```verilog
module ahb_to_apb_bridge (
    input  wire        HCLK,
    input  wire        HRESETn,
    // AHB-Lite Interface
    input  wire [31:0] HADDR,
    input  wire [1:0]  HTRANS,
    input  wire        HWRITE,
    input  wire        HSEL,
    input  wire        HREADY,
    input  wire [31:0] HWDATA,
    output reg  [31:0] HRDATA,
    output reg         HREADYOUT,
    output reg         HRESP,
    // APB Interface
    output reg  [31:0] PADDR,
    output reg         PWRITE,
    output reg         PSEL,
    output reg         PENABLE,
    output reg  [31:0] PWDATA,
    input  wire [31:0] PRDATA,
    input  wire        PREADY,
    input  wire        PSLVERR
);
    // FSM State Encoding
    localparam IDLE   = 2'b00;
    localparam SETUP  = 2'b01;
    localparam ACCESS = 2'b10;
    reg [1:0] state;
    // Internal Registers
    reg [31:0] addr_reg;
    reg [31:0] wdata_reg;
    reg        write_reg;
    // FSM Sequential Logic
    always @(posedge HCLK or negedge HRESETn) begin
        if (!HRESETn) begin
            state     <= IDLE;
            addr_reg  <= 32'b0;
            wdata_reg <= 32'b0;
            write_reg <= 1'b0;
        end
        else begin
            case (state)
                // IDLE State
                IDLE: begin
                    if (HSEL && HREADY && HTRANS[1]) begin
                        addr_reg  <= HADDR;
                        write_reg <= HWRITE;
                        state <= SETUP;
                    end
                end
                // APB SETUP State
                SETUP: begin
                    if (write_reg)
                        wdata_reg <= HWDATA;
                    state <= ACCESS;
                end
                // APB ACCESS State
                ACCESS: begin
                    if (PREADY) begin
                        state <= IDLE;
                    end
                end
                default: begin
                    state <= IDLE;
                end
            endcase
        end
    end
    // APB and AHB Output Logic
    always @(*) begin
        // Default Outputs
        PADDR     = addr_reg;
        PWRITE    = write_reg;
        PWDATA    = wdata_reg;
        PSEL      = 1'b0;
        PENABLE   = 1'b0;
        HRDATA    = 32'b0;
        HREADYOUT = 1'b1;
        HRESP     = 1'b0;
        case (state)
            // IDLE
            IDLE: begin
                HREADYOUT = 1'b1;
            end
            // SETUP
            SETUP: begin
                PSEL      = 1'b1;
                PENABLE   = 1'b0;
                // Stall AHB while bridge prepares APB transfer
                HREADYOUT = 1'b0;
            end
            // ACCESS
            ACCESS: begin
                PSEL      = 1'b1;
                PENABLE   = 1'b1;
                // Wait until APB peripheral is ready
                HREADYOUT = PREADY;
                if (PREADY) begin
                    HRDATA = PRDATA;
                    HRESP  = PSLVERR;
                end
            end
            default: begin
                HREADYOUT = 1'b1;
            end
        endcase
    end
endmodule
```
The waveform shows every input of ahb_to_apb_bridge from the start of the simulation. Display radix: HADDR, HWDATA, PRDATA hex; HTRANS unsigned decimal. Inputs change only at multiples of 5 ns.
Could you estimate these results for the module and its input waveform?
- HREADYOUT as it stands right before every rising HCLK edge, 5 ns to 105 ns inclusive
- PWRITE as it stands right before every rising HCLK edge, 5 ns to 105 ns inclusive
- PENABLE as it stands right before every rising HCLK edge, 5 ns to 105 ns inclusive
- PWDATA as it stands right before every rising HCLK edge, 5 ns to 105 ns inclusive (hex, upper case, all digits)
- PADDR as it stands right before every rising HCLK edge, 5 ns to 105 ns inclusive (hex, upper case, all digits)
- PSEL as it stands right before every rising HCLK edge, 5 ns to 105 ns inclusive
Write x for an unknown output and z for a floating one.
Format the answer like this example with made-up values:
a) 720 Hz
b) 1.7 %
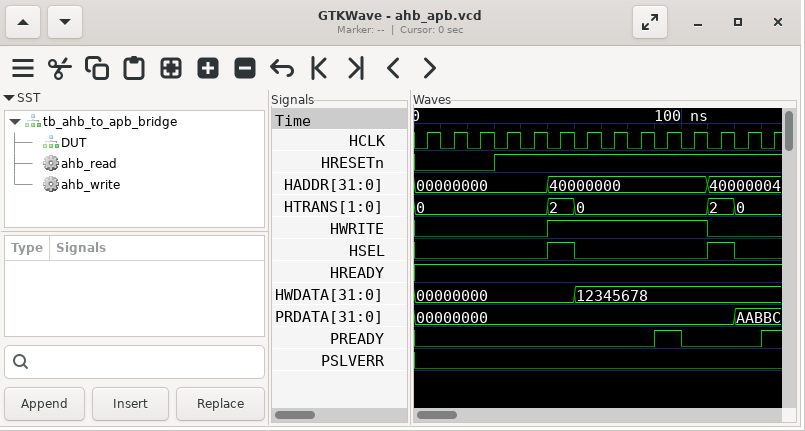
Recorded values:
a) 1 1 1 1 1 1 0 0 0 1 1
b) 0 0 0 0 0 0 1 1 1 1 1
c) 0 0 0 0 0 0 0 1 1 1 0
d) 00000000, 00000000, 00000000, 00000000, 00000000, 00000000, 00000000, 12345678, 12345678, 12345678, 12345678
e) 00000000, 00000000, 00000000, 00000000, 00000000, 00000000, 40000000, 40000000, 40000000, 40000000, 40000000
f) 0 0 0 0 0 0 1 1 1 1 0
